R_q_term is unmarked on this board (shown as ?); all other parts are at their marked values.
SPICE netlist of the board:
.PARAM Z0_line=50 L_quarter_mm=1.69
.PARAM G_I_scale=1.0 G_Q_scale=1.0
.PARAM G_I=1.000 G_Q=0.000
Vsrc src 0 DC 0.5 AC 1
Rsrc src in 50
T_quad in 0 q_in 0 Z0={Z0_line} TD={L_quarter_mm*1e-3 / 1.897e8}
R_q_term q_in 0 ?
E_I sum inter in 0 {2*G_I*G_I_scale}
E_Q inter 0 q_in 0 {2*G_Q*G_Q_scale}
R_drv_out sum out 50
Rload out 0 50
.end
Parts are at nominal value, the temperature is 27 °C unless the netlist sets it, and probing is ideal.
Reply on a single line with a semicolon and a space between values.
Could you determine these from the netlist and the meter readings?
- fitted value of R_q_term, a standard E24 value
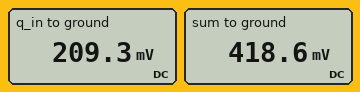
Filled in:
36 Ω
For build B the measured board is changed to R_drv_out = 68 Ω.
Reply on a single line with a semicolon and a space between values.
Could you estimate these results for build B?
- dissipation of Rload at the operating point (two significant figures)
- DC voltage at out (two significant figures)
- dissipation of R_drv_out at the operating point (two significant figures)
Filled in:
630 µW; 180 mV; 860 µW
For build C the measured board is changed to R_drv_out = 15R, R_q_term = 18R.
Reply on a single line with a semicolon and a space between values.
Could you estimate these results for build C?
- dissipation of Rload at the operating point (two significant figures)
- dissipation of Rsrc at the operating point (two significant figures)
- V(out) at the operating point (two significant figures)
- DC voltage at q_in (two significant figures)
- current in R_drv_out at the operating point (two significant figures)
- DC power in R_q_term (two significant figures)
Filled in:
830 µW; 2.7 mW; 200 mV; 130 mV; 4.1 mA; 970 µW
